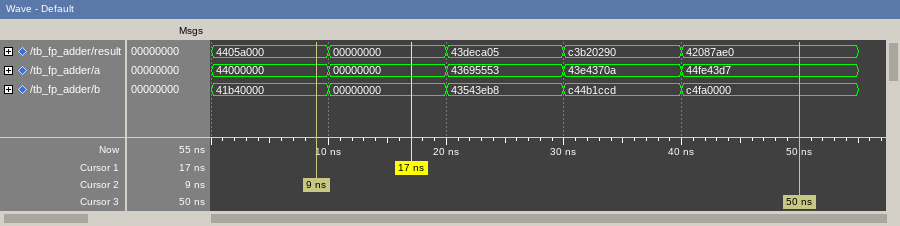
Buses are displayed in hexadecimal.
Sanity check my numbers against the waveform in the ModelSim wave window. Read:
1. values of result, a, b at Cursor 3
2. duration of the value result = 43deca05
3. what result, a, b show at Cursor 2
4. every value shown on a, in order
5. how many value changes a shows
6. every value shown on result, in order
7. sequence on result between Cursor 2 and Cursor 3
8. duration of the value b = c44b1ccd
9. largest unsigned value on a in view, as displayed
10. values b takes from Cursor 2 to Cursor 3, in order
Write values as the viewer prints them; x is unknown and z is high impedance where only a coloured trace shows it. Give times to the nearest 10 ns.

result=42087ae0, a=44fe43d7, b=c4fa0000
10 ns
result=4405a000, a=44000000, b=41b40000
44000000, 00000000, 43695553, 43e4370a, 44fe43d7
4
4405a000, 00000000, 43deca05, c3b20290, 42087ae0
4405a000, 00000000, 43deca05, c3b20290, 42087ae0
10 ns
44fe43d7
41b40000, 00000000, 43543eb8, c44b1ccd, c4fa0000
